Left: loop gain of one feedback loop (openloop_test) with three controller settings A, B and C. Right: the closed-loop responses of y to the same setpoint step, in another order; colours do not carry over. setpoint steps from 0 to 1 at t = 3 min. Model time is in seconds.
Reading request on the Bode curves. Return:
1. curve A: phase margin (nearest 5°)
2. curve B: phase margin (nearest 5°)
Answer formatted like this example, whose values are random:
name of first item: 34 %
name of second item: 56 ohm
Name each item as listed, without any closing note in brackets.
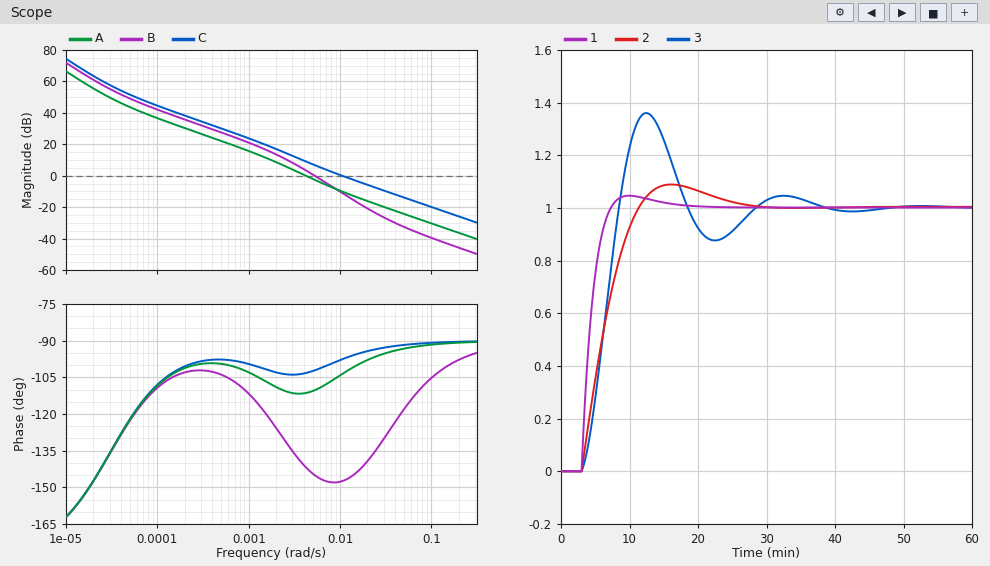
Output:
curve A: phase margin: 70°
curve B: phase margin: 35°
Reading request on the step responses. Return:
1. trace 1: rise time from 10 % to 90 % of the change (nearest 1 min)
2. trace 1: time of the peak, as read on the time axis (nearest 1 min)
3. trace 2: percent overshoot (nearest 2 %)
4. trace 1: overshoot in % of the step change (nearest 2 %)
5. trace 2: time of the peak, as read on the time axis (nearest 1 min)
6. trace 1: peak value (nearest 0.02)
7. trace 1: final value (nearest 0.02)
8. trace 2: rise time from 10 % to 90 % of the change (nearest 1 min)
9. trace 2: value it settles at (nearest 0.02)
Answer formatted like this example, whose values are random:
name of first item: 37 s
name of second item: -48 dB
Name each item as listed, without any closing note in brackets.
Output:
trace 1: rise time from 10 % to 90 % of the change: 3 min
trace 1: time of the peak, as read on the time axis: 10 min
trace 2: percent overshoot: 8 %
trace 1: overshoot in % of the step change: 4 %
trace 2: time of the peak, as read on the time axis: 16 min
trace 1: peak value: 1.04
trace 1: final value: 1.00
trace 2: rise time from 10 % to 90 % of the change: 6 min
trace 2: value it settles at: 1.00
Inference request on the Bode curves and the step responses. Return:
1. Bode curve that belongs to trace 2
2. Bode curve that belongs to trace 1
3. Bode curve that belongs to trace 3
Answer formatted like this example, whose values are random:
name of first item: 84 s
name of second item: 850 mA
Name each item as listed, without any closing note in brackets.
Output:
Bode curve that belongs to trace 2: A
Bode curve that belongs to trace 1: C
Bode curve that belongs to trace 3: B
